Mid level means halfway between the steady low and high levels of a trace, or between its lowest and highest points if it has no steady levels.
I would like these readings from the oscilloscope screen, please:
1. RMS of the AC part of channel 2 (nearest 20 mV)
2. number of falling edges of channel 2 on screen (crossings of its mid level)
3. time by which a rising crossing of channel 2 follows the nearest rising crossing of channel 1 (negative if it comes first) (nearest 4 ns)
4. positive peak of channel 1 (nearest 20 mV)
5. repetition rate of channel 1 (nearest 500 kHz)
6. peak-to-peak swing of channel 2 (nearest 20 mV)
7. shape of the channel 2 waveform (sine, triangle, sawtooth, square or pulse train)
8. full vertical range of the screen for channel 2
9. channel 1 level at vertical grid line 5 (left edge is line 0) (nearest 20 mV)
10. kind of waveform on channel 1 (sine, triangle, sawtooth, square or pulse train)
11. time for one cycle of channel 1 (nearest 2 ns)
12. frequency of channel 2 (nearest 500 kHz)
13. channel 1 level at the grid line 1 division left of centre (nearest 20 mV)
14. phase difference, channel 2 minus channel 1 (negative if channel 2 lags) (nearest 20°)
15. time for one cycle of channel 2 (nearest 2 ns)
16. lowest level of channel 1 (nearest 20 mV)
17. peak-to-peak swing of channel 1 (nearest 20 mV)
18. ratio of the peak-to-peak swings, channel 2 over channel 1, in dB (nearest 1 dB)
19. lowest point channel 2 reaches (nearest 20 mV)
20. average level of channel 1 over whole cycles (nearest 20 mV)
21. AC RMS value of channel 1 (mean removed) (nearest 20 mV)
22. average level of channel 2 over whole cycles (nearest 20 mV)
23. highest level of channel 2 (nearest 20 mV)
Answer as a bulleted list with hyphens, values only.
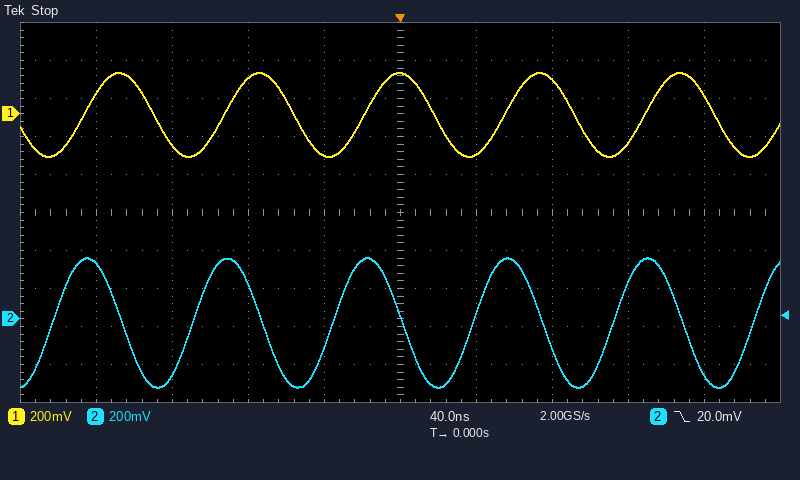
- 240 mV
- 5
- -16 ns
- 220 mV
- 13.5 MHz
- 680 mV
- sine
- 2 V
- 220 mV
- sine
- 74 ns
- 13.5 MHz
- -220 mV
- +80°
- 74 ns
- -220 mV
- 440 mV
- 4 dB
- -360 mV
- 0 mV
- 160 mV
- -20 mV
- 320 mV
